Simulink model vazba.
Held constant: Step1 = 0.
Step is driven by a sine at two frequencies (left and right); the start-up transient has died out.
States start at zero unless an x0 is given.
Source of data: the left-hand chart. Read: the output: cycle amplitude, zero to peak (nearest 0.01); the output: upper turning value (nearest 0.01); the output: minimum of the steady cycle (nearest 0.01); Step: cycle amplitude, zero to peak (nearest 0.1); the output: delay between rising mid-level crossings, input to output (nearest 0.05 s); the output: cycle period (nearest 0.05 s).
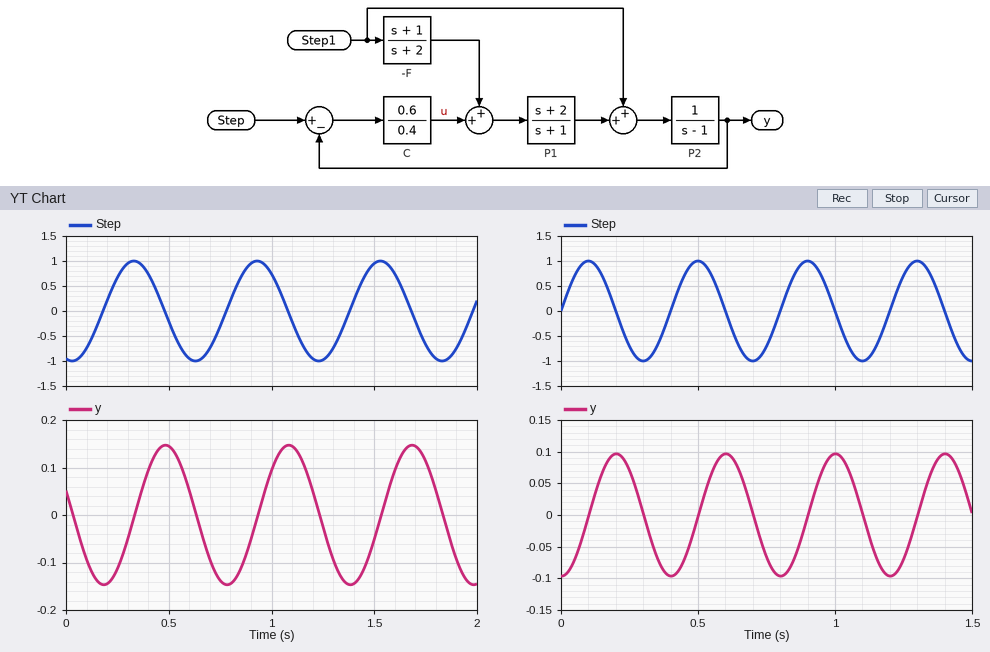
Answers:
0.15
0.15
-0.15
1.0
0.15 s
0.60 s
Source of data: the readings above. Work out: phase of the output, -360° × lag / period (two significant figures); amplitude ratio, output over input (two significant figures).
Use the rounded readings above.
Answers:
-90°
0.15
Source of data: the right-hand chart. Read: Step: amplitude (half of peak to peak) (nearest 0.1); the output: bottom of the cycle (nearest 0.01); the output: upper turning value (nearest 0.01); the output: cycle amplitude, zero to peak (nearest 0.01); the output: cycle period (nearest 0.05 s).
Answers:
1.0
-0.10
0.10
0.10
0.40 s
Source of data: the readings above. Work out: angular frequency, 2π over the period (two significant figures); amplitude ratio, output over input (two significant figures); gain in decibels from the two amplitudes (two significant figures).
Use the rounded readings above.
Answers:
16 rad/s
0.10
-20 dB
